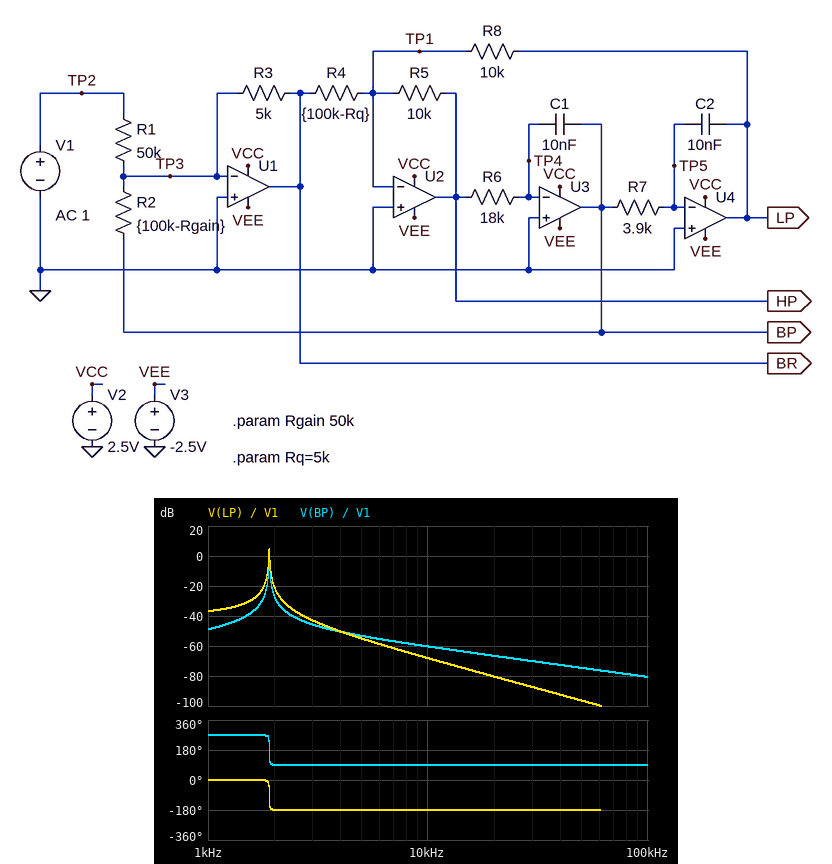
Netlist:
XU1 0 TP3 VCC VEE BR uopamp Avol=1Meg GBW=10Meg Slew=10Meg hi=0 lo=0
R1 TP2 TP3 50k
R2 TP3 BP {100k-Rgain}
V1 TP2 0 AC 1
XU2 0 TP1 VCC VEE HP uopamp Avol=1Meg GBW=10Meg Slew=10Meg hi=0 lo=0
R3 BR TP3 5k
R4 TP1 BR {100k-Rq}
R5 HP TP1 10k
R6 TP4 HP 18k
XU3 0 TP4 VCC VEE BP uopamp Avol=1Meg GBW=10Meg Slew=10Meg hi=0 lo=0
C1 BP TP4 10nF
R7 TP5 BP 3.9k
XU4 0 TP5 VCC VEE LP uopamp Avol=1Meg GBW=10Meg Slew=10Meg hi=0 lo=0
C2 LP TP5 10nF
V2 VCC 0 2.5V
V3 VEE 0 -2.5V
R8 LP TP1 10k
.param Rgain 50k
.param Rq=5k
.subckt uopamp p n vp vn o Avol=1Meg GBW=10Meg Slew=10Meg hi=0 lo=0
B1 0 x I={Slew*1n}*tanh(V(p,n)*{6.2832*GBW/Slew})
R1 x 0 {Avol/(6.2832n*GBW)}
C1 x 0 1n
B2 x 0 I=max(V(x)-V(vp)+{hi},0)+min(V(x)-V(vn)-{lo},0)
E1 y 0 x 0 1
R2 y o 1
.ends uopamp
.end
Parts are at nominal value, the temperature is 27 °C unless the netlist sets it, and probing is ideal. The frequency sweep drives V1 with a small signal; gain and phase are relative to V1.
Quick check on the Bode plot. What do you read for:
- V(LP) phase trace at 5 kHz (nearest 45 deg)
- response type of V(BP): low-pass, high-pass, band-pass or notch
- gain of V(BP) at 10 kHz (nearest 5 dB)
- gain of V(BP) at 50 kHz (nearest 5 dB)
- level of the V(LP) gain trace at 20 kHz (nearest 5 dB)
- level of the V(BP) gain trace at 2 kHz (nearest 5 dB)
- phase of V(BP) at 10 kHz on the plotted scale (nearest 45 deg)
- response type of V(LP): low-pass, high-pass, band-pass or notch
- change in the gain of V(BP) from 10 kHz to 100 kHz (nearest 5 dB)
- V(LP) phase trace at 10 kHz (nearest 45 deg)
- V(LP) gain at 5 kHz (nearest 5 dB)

-180 deg
band-pass
-60 dB
-75 dB
-80 dB
-25 dB
90 deg
band-pass
-20 dB
-180 deg
-55 dB
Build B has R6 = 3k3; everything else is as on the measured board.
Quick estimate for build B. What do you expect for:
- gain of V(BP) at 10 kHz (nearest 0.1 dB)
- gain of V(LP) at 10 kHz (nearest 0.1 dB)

-44.0 dB
-51.8 dB
